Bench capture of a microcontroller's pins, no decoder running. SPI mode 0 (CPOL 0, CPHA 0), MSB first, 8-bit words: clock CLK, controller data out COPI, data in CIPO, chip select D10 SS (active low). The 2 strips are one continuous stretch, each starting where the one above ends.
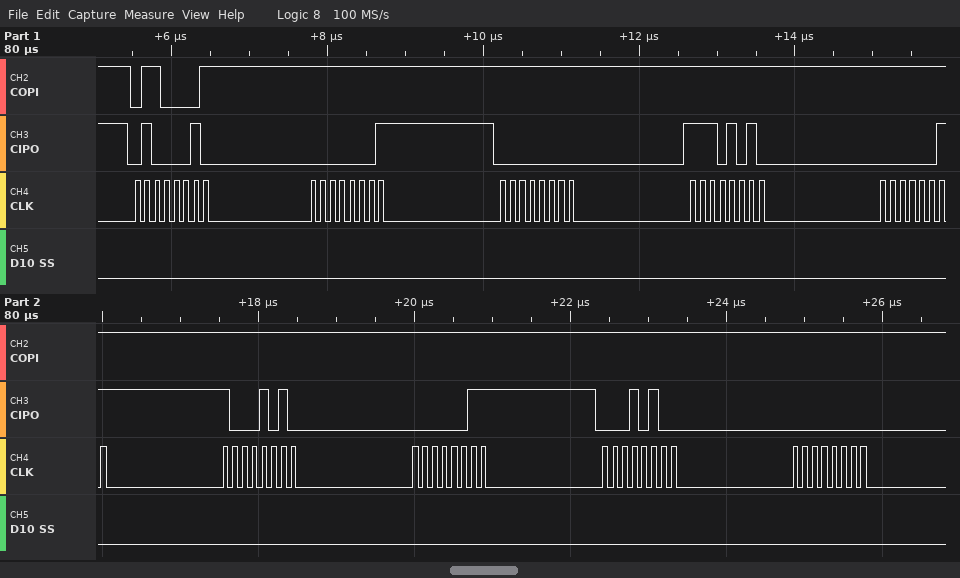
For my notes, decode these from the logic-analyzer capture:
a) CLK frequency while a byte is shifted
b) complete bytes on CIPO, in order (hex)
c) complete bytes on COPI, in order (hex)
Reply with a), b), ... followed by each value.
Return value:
a) 8 MHz
b) 42 01 00 EA 03 8A 03 14 00
c) 61 FF FF FF FF FF FF FF FF
